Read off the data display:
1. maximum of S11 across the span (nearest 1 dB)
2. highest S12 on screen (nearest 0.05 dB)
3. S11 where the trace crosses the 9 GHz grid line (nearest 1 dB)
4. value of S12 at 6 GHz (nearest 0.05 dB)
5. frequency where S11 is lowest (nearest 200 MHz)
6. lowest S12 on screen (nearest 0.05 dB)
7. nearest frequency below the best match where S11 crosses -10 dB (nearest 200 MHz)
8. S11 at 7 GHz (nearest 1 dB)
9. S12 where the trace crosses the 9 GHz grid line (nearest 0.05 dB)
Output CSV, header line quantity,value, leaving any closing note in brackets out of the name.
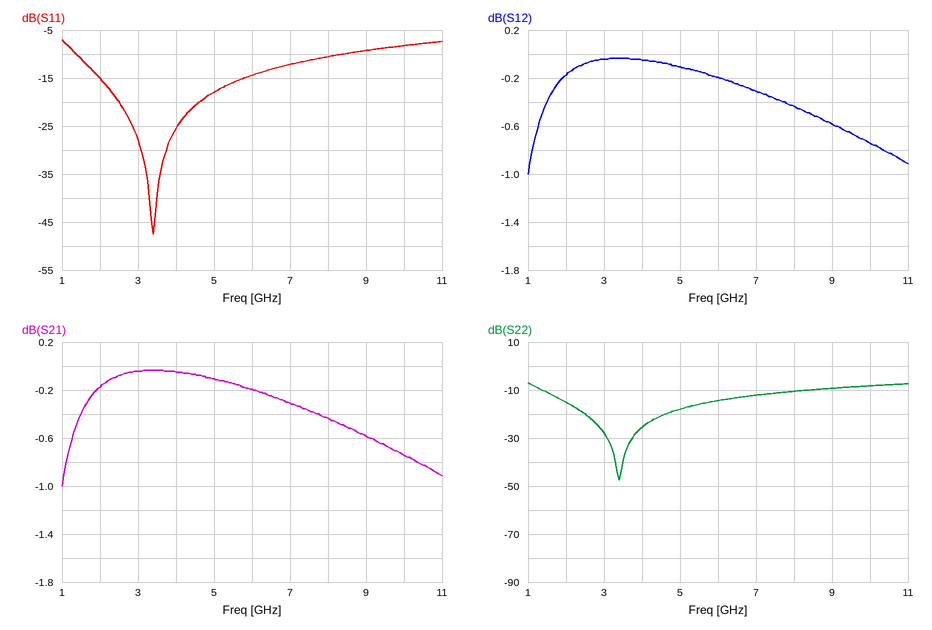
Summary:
quantity,value
maximum of S11 across the span,-7 dB
highest S12 on screen,-0.05 dB
S11 where the trace crosses the 9 GHz grid line,-9 dB
value of S12 at 6 GHz,-0.20 dB
frequency where S11 is lowest,3.4 GHz
lowest S12 on screen,-1.00 dB
nearest frequency below the best match where S11 crosses -10 dB,1.4 GHz
S11 at 7 GHz,-12 dB
S12 where the trace crosses the 9 GHz grid line,-0.60 dB
